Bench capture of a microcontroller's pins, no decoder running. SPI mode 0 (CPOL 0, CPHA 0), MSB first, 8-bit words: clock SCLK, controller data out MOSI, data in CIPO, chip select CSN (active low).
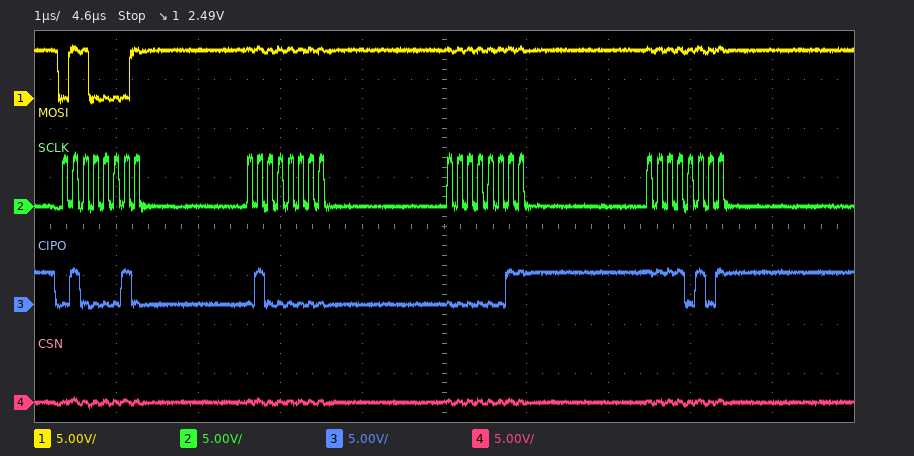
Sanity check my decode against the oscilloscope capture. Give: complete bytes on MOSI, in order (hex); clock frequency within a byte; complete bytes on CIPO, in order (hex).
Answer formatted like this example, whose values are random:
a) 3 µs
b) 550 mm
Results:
a) 0x61 0xFF 0xFF 0xFF
b) 8 MHz
c) 0x42 0x40 0x03 0xF5
